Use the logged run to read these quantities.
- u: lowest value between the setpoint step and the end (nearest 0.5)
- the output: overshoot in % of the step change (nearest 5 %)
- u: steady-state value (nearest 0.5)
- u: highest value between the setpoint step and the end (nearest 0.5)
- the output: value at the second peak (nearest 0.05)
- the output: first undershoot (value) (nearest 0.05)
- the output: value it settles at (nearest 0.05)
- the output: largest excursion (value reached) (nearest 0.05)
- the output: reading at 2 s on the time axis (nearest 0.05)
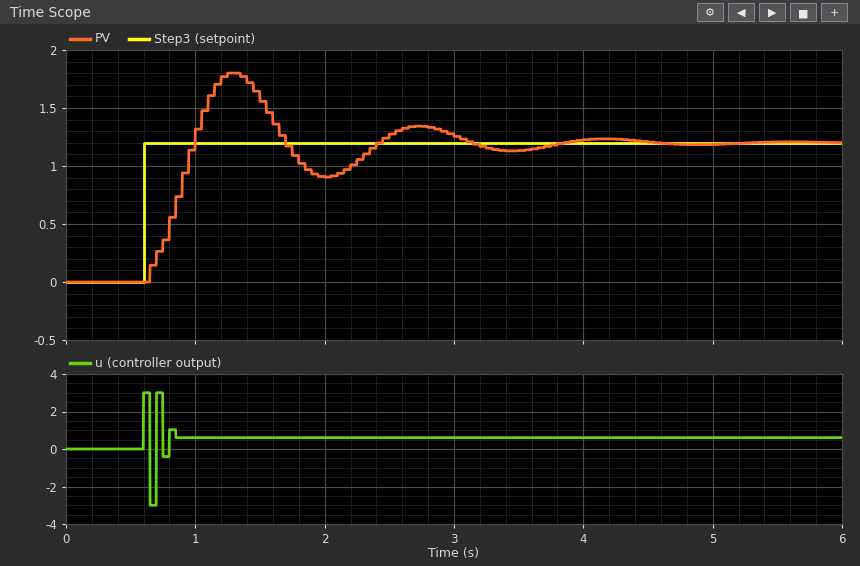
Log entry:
-3.0
50 %
0.5
3.0
1.35
0.90
1.20
1.80
0.90
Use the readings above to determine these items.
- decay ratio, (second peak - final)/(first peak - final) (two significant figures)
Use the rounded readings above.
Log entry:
0.25
